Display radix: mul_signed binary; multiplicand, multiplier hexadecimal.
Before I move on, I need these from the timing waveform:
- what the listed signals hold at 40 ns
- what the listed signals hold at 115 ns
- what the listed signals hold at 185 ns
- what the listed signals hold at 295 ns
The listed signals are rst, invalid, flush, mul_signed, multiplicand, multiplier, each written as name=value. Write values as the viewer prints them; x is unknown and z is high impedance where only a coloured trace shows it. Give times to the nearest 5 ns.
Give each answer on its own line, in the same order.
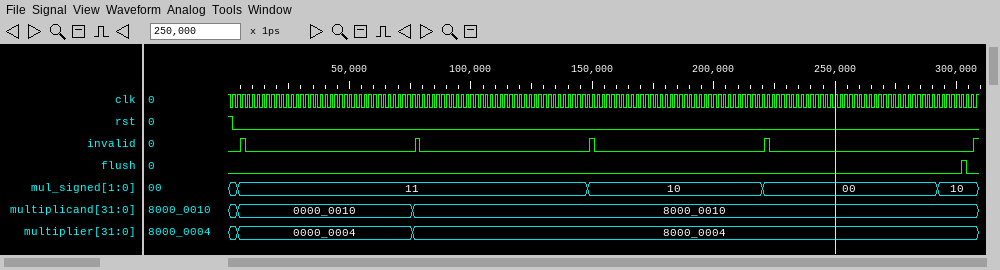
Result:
rst=0, invalid=0, flush=0, mul_signed=11, multiplicand=0000_0010, multiplier=0000_0004
rst=0, invalid=0, flush=0, mul_signed=11, multiplicand=8000_0010, multiplier=8000_0004
rst=0, invalid=0, flush=0, mul_signed=10, multiplicand=8000_0010, multiplier=8000_0004
rst=0, invalid=0, flush=0, mul_signed=10, multiplicand=8000_0010, multiplier=8000_0004
